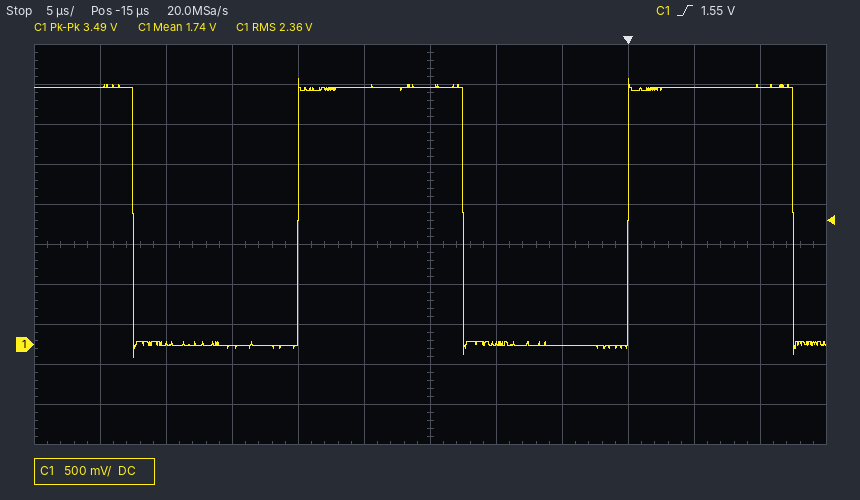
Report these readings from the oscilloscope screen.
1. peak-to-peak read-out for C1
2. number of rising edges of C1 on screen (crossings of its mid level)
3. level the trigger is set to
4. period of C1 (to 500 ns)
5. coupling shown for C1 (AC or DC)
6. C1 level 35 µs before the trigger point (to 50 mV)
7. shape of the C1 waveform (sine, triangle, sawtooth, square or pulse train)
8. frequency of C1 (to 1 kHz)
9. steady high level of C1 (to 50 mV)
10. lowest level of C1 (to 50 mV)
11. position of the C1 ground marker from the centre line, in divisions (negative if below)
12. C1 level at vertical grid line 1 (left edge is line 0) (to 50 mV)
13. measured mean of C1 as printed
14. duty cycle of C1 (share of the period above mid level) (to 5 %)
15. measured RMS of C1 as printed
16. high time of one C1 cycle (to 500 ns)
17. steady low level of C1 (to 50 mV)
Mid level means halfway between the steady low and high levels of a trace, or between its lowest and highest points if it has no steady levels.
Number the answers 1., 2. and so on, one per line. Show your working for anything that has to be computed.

1. 3.49 V
2. 2
3. 1.55 V
4. 25.0 µs
5. DC
6. 0 mV
7. square
8. 1 / 25.0 µs ≈ 40 kHz
9. 3.20 V
10. -150 mV
11. -2.5 div
12. 3.20 V
13. 1.74 V
14. 12.5 µs / 25.0 µs ≈ 50 %
15. 2.36 V
16. 12.5 µs
17. 0 mV
